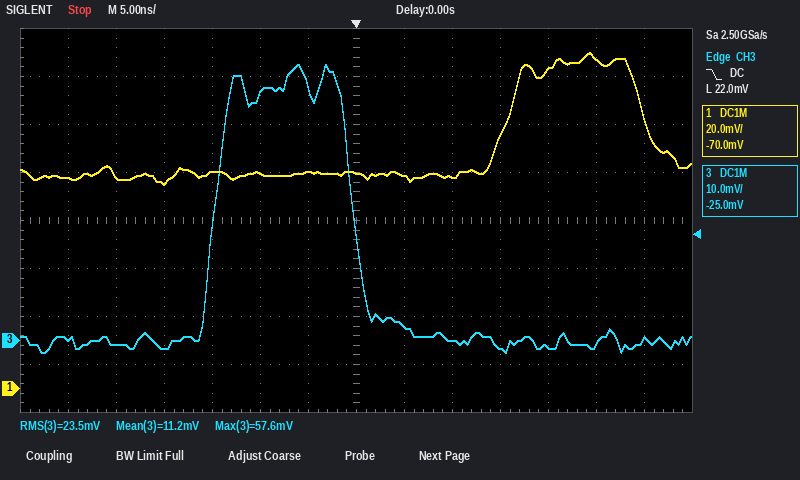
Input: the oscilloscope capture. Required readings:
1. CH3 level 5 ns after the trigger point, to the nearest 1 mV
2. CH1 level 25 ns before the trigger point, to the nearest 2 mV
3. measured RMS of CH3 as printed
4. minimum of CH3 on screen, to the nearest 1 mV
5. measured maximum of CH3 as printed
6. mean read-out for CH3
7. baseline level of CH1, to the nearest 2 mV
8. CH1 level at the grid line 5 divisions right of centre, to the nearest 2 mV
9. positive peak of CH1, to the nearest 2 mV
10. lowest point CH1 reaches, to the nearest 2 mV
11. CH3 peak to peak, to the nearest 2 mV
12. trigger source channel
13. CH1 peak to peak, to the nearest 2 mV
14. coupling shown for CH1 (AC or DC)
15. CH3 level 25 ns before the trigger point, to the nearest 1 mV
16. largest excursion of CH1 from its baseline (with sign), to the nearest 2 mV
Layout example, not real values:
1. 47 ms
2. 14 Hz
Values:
1. 3 mV
2. 88 mV
3. 23.5 mV
4. -2 mV
5. 57.6 mV
6. 11.2 mV
7. 90 mV
8. 138 mV
9. 140 mV
10. 84 mV
11. 60 mV
12. CH3
13. 56 mV
14. DC
15. -1 mV
16. +50 mV
